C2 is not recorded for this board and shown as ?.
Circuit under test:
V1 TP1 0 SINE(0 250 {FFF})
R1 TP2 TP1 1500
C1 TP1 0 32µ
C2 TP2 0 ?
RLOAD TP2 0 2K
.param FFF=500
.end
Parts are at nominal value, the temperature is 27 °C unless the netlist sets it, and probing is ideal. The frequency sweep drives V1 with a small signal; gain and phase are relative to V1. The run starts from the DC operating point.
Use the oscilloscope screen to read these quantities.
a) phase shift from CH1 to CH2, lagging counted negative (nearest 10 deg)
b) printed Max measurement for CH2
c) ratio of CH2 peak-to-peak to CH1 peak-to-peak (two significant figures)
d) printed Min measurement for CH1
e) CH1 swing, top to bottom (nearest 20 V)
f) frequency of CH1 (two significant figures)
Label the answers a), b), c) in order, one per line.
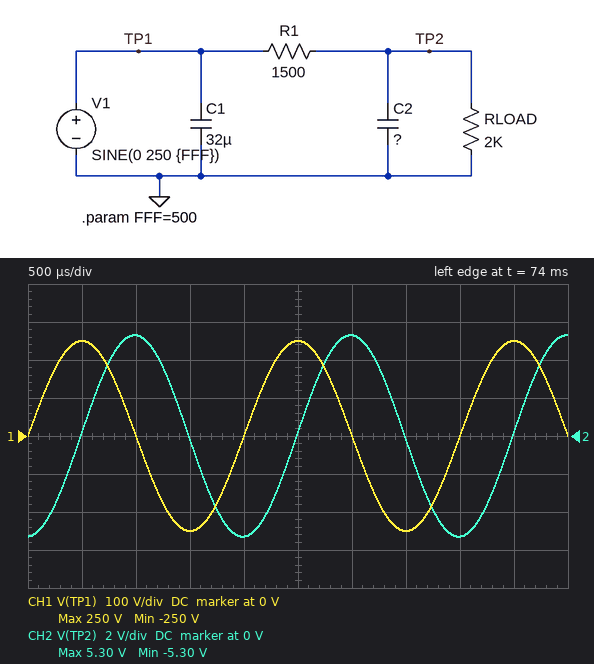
a) -90 deg
b) 5.30 V
c) 0.021
d) -250 V
e) 500 V
f) 500 Hz
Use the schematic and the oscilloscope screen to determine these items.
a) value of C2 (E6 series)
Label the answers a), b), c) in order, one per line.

a) 10 µF
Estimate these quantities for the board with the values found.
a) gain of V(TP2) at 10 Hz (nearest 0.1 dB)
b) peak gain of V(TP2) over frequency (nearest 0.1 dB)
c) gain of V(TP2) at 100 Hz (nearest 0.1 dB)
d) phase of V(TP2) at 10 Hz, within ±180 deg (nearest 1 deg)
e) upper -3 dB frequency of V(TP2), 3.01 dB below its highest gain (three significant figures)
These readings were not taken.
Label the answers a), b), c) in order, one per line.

a) -6.0 dB
b) -4.9 dB
c) -19.6 dB
d) -28 deg
e) 18.6 Hz
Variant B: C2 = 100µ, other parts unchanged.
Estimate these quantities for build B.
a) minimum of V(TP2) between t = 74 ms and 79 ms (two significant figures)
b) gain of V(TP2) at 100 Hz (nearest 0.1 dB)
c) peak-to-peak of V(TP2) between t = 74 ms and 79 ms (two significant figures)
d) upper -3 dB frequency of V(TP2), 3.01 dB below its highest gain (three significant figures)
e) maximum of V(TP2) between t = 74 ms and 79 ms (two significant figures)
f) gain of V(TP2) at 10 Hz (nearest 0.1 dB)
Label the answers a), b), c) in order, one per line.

a) -320 mV
b) -39.5 dB
c) 1.1 V
d) 1.86 Hz
e) 750 mV
f) -19.6 dB
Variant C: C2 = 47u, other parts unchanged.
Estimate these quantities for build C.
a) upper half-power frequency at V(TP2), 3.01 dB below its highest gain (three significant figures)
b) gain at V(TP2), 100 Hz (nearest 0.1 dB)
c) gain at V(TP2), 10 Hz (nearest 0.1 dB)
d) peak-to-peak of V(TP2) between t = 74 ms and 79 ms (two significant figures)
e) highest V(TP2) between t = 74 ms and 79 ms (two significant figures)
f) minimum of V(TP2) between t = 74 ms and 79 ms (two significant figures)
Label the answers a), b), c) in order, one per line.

a) 3.95 Hz
b) -32.9 dB
c) -13.6 dB
d) 2.3 V
e) 1.3 V
f) -970 mV
